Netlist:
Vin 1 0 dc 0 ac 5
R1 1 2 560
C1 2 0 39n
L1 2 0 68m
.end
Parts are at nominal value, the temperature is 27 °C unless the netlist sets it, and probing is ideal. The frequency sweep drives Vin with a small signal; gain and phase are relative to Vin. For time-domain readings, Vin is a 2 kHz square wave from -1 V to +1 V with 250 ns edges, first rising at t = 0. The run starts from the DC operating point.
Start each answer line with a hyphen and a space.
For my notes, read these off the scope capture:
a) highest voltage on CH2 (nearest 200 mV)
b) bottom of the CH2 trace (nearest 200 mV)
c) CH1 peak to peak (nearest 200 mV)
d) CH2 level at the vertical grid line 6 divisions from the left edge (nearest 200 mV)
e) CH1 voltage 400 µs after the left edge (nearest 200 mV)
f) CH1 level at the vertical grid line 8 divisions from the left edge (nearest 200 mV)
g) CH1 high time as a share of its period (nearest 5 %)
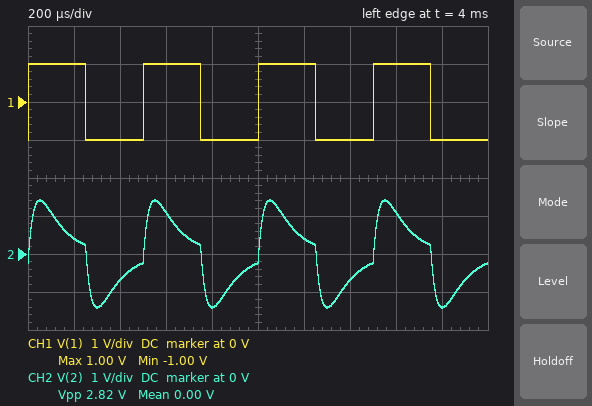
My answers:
- 1.4 V
- -1.4 V
- 2.0 V
- 400 mV
- -1.0 V
- 1.0 V
- 50 %
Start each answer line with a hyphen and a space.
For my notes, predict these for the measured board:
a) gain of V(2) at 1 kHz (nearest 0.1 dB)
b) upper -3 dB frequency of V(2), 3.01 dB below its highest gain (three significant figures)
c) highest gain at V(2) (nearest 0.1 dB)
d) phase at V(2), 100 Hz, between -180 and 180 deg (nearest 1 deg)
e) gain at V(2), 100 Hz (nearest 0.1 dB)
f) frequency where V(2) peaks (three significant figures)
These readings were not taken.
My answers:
- -3.8 dB
- 8.42 kHz
- 0 dB
- 86 deg
- -22.4 dB
- 3.09 kHz
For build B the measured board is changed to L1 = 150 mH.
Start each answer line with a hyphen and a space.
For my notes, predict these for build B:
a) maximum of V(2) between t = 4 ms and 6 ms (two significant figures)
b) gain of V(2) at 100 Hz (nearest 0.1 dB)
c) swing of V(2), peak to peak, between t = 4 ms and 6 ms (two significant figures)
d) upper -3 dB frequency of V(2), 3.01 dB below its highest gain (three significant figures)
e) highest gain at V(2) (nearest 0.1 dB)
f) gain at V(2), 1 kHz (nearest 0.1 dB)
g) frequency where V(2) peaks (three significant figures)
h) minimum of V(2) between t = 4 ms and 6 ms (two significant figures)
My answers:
- 1.2 V
- -15.6 dB
- 2.4 V
- 7.84 kHz
- 0 dB
- -0.8 dB
- 2.08 kHz
- -1.2 V
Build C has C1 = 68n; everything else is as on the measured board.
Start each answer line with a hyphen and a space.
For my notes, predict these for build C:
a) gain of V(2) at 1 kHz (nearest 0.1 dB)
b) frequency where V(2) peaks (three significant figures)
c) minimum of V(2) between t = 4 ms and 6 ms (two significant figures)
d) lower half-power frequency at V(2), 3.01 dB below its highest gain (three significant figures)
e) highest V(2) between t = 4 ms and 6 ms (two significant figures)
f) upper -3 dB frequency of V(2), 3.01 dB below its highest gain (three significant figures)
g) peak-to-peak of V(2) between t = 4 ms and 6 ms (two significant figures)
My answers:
- -3.3 dB
- 2.34 kHz
- -1.3 V
- 1.05 kHz
- 1.3 V
- 5.23 kHz
- 2.6 V
